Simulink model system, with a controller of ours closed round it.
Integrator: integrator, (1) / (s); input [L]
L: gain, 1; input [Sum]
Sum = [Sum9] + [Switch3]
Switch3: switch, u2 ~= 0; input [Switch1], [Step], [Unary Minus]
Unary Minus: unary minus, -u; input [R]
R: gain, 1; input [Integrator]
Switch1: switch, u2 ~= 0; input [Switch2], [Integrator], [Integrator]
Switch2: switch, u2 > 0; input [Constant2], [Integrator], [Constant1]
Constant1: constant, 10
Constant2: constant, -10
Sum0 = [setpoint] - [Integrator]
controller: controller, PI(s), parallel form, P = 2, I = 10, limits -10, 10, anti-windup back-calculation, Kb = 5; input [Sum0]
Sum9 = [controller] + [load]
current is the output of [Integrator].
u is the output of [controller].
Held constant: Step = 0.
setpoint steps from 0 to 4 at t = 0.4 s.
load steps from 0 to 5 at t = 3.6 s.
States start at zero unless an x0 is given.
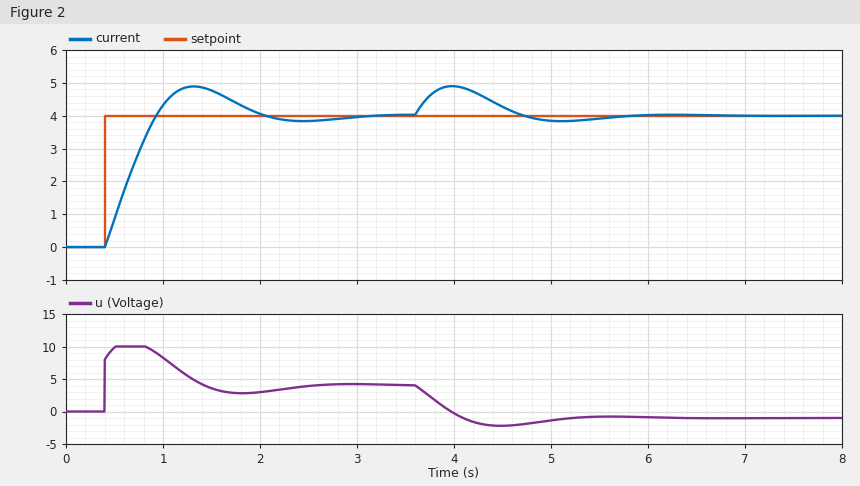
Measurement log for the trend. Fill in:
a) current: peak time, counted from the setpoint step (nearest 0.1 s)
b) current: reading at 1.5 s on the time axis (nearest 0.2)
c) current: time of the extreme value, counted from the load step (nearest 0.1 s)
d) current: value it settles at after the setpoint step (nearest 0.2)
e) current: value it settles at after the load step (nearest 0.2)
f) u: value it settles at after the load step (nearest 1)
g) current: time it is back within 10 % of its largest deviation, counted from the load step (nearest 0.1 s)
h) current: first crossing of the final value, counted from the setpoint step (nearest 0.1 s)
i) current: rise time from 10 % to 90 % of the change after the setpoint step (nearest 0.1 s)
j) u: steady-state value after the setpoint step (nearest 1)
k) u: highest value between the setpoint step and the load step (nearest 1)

0.9 s
4.8
0.4 s
4.0
4.0
-1
1.9 s
0.5 s
0.4 s
4
10
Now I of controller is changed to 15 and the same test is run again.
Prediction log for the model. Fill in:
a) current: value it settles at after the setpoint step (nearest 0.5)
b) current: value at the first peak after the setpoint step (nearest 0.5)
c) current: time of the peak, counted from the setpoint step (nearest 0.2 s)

4.0
5.0
0.8 s
